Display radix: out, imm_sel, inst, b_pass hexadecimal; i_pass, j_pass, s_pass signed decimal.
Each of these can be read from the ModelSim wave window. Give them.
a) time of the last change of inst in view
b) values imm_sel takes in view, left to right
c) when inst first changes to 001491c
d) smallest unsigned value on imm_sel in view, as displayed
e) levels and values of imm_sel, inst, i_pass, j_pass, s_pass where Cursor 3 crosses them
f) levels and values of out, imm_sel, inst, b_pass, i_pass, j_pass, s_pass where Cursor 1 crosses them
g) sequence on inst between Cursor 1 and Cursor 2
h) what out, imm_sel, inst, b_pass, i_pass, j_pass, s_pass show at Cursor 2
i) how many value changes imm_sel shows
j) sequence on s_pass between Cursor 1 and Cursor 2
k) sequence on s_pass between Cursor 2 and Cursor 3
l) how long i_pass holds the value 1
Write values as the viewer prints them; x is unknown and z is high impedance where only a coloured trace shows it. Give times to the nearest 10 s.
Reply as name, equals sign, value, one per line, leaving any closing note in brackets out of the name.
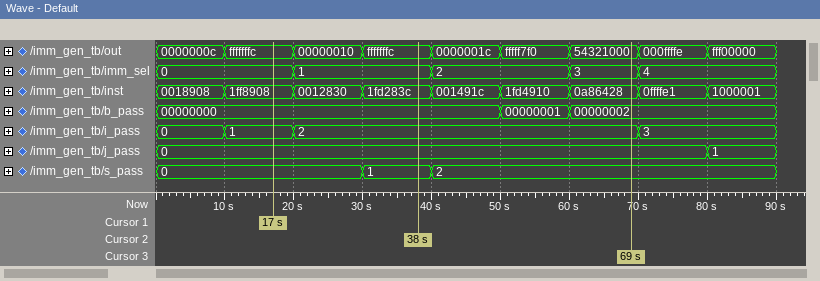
time of the last change of inst in view = 80 s
values imm_sel takes in view, left to right = 0, 1, 2, 3, 4
when inst first changes to 001491c = 40 s
smallest unsigned value on imm_sel in view, as displayed = 0
levels and values of imm_sel, inst, i_pass, j_pass, s_pass where Cursor 3 crosses them = imm_sel=3, inst=0a86428, i_pass=2, j_pass=0, s_pass=2
levels and values of out, imm_sel, inst, b_pass, i_pass, j_pass, s_pass where Cursor 1 crosses them = out=fffffffc, imm_sel=0, inst=1ff8908, b_pass=00000000, i_pass=1, j_pass=0, s_pass=0
sequence on inst between Cursor 1 and Cursor 2 = 1ff8908, 0012830, 1fd283c
what out, imm_sel, inst, b_pass, i_pass, j_pass, s_pass show at Cursor 2 = out=fffffffc, imm_sel=1, inst=1fd283c, b_pass=00000000, i_pass=2, j_pass=0, s_pass=1
how many value changes imm_sel shows = 4
sequence on s_pass between Cursor 1 and Cursor 2 = 0, 1
sequence on s_pass between Cursor 2 and Cursor 3 = 1, 2
how long i_pass holds the value 1 = 10 s
